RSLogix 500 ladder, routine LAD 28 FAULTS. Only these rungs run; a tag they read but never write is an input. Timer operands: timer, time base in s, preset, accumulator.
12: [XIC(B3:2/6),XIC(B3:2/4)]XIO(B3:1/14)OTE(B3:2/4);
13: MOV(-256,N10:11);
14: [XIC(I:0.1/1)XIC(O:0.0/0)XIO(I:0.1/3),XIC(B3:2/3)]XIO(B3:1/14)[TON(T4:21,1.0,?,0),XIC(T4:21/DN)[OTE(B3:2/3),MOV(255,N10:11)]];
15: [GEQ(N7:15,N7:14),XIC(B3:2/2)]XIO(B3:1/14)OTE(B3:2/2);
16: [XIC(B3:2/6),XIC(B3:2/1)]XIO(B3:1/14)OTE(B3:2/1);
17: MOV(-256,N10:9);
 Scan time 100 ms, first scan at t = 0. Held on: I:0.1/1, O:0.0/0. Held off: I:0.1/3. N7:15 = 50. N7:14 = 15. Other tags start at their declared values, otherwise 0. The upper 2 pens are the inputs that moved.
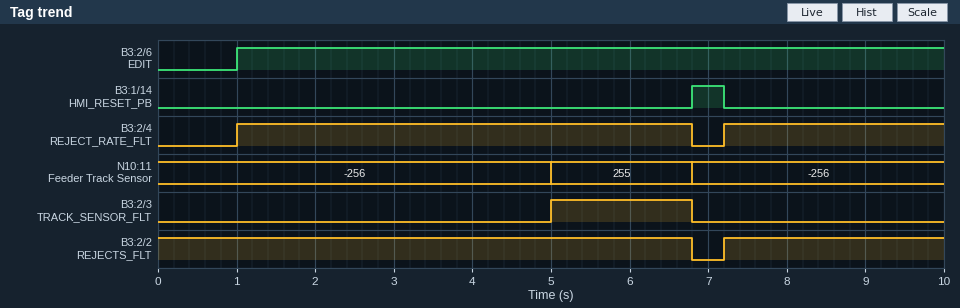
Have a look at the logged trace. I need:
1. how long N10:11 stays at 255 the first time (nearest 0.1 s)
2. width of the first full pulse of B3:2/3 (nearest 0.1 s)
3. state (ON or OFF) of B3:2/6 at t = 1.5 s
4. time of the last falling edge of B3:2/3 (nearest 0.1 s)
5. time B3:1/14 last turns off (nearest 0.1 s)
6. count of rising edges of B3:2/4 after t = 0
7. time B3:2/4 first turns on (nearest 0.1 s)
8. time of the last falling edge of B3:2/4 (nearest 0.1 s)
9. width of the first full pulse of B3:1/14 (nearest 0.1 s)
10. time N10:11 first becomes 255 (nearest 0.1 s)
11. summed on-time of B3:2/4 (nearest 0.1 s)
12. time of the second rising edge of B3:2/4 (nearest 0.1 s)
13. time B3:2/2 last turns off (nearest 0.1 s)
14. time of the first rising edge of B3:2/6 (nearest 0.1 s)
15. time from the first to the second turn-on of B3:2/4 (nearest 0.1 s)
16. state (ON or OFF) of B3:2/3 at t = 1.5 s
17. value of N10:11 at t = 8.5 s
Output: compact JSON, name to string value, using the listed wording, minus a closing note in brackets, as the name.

{"how long N10:11 stays at 255 the first time": "1.8 s", "width of the first full pulse of B3:2/3": "1.8 s", "state (ON or OFF) of B3:2/6 at t = 1.5 s": "ON", "time of the last falling edge of B3:2/3": "6.8 s", "time B3:1/14 last turns off": "7.2 s", "count of rising edges of B3:2/4 after t = 0": "2", "time B3:2/4 first turns on": "1.0 s", "time of the last falling edge of B3:2/4": "6.8 s", "width of the first full pulse of B3:1/14": "0.4 s", "time N10:11 first becomes 255": "5.0 s", "summed on-time of B3:2/4": "8.6 s", "time of the second rising edge of B3:2/4": "7.2 s", "time B3:2/2 last turns off": "6.8 s", "time of the first rising edge of B3:2/6": "1.0 s", "time from the first to the second turn-on of B3:2/4": "6.2 s", "state (ON or OFF) of B3:2/3 at t = 1.5 s": "OFF", "value of N10:11 at t = 8.5 s": "-256"}
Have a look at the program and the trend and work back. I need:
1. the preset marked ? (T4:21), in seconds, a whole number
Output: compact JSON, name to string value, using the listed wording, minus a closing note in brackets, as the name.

{"the preset marked ? (T4:21), in seconds, a whole number": "5 s"}
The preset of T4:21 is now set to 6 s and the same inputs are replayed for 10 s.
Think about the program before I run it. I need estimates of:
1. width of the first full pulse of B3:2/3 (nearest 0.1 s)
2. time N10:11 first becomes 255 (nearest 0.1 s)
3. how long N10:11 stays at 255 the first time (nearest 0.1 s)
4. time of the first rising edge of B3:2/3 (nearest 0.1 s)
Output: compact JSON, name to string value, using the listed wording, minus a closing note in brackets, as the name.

{"width of the first full pulse of B3:2/3": "0.8 s", "time N10:11 first becomes 255": "6.0 s", "how long N10:11 stays at 255 the first time": "0.8 s", "time of the first rising edge of B3:2/3": "6.0 s"}
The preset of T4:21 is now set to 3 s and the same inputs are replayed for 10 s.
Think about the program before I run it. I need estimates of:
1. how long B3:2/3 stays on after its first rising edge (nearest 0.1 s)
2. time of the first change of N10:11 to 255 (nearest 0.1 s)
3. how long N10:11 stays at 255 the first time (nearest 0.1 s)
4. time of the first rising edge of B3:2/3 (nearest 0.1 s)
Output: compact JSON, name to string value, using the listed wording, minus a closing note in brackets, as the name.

{"how long B3:2/3 stays on after its first rising edge": "3.8 s", "time of the first change of N10:11 to 255": "3.0 s", "how long N10:11 stays at 255 the first time": "3.8 s", "time of the first rising edge of B3:2/3": "3.0 s"}
